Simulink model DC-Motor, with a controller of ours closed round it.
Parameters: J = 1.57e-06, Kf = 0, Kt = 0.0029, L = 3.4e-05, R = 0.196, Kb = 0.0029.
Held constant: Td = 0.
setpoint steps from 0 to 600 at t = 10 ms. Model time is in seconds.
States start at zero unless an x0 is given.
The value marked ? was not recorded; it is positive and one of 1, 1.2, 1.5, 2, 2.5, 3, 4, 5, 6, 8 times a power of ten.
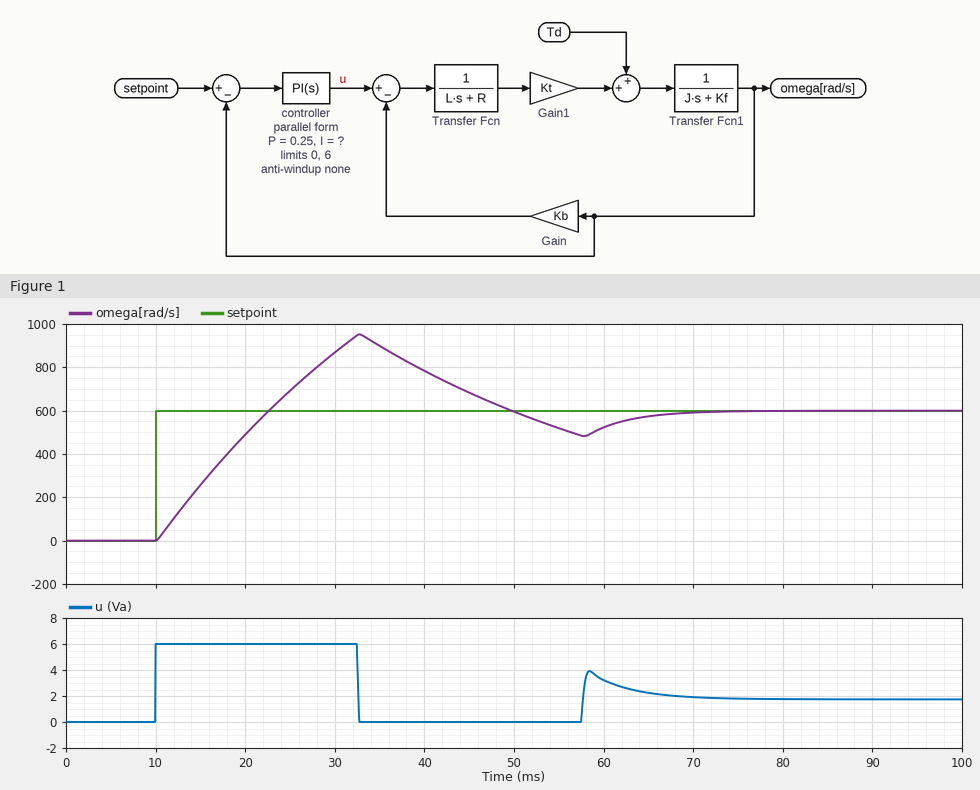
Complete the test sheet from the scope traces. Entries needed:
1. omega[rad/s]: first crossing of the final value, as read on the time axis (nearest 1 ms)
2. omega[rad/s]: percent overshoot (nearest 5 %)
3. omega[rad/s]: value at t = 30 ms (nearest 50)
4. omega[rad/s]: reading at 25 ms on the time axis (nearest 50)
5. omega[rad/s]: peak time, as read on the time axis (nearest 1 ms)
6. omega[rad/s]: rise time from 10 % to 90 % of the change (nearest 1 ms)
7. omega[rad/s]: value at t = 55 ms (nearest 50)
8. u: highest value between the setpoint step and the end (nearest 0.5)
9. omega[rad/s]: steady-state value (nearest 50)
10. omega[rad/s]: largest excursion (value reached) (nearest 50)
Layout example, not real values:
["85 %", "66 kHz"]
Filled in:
["23 ms", "60 %", "850", "700", "33 ms", "10 ms", "500", "6.0", "600", "950"]
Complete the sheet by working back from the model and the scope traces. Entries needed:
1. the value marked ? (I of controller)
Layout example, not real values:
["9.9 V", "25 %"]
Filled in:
["50"]
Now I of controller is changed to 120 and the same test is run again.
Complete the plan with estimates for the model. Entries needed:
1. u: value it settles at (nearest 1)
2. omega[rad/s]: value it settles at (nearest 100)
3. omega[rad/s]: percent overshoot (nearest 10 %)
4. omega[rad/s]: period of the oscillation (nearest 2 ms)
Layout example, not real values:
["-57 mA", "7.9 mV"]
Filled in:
["2", "600", "70 %", "46 ms"]
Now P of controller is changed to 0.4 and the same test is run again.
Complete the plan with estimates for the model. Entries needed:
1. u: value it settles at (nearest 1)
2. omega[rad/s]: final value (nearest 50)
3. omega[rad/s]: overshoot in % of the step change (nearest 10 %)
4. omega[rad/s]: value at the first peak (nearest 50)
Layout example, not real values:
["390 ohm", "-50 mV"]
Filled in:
["2", "600", "50 %", "900"]
